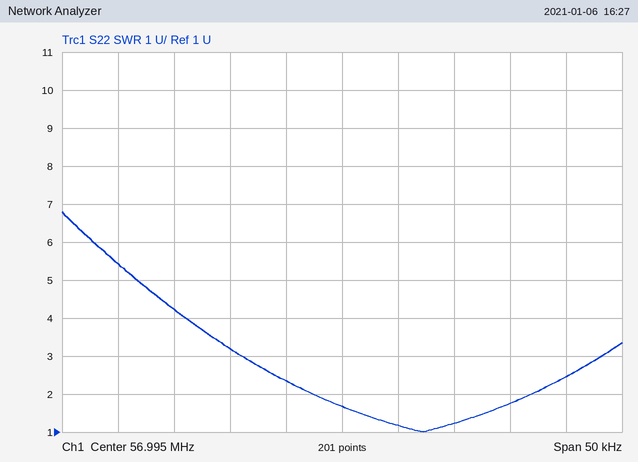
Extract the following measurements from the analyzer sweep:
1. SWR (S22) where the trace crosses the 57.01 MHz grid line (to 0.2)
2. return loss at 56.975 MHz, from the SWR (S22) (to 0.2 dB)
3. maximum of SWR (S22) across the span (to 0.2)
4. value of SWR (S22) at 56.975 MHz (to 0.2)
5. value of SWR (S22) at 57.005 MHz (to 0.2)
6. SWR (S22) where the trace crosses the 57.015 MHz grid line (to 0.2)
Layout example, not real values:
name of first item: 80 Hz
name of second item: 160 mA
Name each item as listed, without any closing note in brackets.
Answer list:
SWR (S22) where the trace crosses the 57.01 MHz grid line: 1.8
return loss at 56.975 MHz, from the SWR (S22): 3.2 dB
maximum of SWR (S22) across the span: 6.8
value of SWR (S22) at 56.975 MHz: 5.4
value of SWR (S22) at 57.005 MHz: 1.2
SWR (S22) where the trace crosses the 57.015 MHz grid line: 2.4
